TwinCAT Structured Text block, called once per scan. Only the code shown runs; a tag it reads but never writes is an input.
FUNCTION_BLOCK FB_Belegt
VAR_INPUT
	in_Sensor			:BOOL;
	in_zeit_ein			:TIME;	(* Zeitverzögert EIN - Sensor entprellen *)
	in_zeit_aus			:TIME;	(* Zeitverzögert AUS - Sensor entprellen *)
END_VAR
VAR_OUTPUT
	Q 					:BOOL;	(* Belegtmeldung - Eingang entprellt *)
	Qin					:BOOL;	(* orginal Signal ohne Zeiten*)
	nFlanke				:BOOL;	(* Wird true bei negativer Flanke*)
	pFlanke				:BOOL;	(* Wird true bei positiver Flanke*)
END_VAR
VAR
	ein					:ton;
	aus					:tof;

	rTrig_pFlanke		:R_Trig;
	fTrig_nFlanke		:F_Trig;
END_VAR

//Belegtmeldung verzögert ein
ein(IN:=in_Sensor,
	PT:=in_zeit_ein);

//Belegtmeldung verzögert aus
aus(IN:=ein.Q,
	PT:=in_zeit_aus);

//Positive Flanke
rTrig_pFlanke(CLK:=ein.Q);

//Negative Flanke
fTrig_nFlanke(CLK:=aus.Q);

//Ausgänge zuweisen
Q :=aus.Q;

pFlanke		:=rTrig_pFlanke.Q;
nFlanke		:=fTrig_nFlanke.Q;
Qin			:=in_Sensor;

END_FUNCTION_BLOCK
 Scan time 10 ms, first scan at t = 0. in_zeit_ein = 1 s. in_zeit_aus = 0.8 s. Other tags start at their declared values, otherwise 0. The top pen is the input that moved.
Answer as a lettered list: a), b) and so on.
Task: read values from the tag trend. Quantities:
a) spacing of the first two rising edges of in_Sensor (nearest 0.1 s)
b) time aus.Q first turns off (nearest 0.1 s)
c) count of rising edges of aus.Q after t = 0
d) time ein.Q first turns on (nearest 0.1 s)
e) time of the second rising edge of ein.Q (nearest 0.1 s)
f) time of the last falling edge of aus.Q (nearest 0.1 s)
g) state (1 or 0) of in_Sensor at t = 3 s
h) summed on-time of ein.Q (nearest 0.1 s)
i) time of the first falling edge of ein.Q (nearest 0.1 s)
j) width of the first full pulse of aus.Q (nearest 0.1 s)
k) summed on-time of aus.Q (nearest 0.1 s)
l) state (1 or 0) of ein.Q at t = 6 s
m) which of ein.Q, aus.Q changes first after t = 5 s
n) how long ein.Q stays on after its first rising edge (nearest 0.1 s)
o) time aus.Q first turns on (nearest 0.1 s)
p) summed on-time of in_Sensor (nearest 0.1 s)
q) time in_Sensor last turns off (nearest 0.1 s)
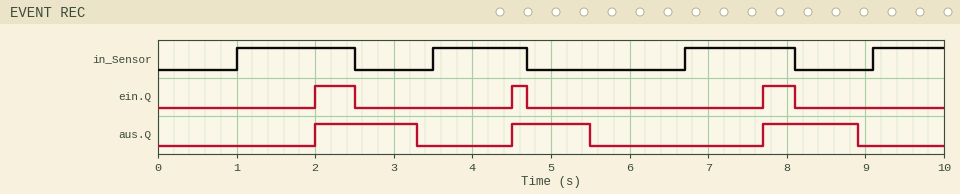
a) 2.5 s
b) 3.3 s
c) 3
d) 2.0 s
e) 4.5 s
f) 8.9 s
g) 0
h) 1.1 s
i) 2.5 s
j) 1.3 s
k) 3.5 s
l) 0
m) aus.Q
n) 0.5 s
o) 2.0 s
p) 5.0 s
q) 8.1 s
